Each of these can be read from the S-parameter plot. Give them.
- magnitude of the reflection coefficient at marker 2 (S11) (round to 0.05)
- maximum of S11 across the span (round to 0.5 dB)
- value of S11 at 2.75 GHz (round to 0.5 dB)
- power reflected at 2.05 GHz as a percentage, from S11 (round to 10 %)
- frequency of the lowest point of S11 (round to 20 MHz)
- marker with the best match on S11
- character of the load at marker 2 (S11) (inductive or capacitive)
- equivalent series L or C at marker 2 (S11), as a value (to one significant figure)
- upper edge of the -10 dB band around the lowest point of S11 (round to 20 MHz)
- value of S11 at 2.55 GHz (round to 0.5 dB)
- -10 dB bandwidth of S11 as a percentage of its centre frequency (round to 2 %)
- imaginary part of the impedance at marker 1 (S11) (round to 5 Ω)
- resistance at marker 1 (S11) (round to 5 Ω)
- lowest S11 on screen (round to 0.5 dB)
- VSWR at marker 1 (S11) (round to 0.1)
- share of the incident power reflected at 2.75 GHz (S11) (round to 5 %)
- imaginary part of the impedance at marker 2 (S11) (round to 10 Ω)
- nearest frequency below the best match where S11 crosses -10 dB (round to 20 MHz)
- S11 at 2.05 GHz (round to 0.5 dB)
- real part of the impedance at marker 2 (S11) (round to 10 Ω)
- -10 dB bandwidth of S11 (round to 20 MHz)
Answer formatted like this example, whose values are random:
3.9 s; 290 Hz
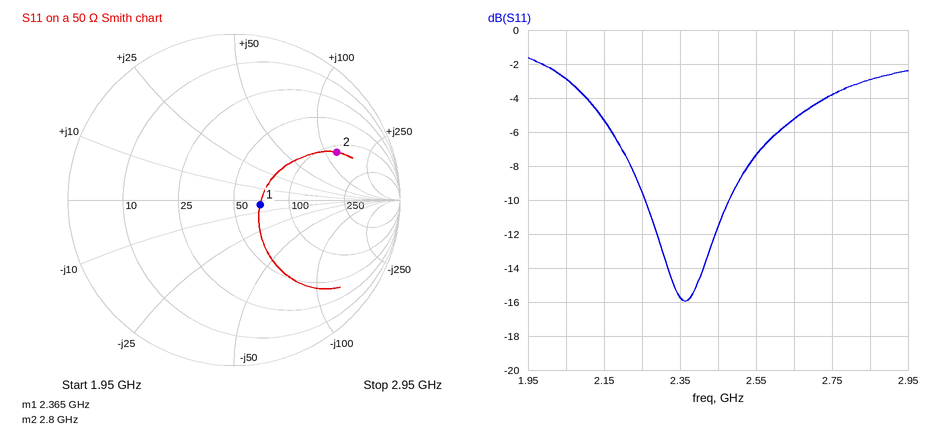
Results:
0.70; -1.5 dB; -4.0 dB; 50 %; 2.36 GHz; marker 1; inductive; 7 nH; 2.48 GHz; -7.5 dB; 10 %; -5 Ω; 70 Ω; -16.0 dB; 1.4; 40 %; +130 Ω; 2.26 GHz; -3.0 dB; 120 Ω; 220 MHz
